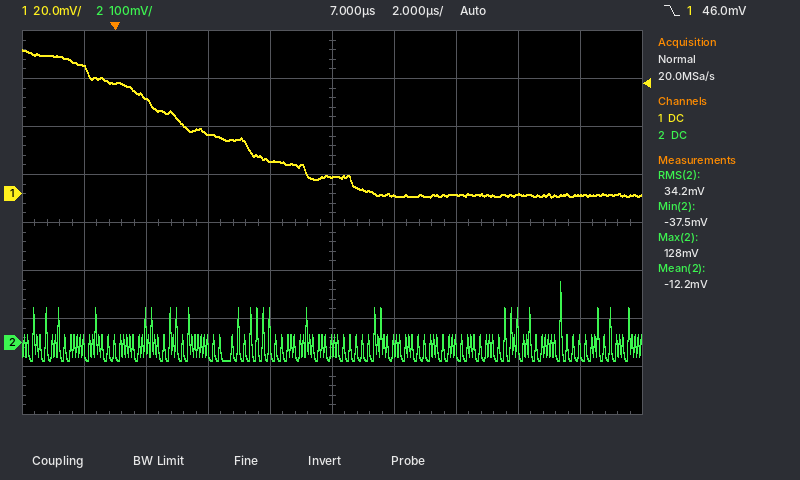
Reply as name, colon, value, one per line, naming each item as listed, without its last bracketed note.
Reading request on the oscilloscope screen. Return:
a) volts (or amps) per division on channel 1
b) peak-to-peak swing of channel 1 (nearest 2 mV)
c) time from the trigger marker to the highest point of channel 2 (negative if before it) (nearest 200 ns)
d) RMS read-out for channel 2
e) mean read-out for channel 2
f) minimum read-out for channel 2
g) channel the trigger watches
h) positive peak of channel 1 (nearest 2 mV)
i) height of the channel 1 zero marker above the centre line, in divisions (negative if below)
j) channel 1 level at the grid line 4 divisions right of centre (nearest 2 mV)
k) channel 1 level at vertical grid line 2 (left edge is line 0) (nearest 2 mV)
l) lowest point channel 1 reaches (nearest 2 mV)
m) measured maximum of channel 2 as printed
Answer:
volts (or amps) per division on channel 1: 20 mV
peak-to-peak swing of channel 1: 62 mV
time from the trigger marker to the highest point of channel 2 (negative if before it): +14.4 µs
RMS read-out for channel 2: 34.2 mV
mean read-out for channel 2: -12.2 mV
minimum read-out for channel 2: -37.5 mV
channel the trigger watches: channel 1
positive peak of channel 1: 60 mV
height of the channel 1 zero marker above the centre line, in divisions: +0.6 div
channel 1 level at the grid line 4 divisions right of centre: 0 mV
channel 1 level at vertical grid line 2 (left edge is line 0): 40 mV
lowest point channel 1 reaches: -2 mV
measured maximum of channel 2 as printed: 128 mV
